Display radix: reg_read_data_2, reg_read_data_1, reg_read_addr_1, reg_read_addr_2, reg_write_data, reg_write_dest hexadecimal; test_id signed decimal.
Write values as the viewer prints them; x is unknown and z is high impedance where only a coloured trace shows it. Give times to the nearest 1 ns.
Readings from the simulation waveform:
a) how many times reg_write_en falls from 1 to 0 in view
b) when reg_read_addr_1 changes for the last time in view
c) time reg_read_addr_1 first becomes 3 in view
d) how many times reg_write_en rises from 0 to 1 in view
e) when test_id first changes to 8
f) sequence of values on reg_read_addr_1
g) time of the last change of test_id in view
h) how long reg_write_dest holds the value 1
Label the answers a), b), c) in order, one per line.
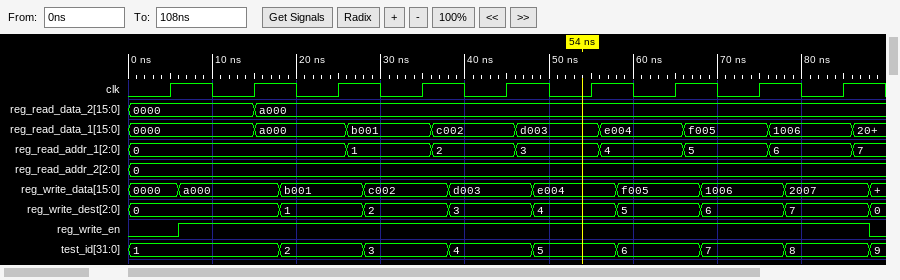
a) 1
b) 86 ns
c) 46 ns
d) 1
e) 78 ns
f) 0, 1, 2, 3, 4, 5, 6, 7
g) 88 ns
h) 10 ns
